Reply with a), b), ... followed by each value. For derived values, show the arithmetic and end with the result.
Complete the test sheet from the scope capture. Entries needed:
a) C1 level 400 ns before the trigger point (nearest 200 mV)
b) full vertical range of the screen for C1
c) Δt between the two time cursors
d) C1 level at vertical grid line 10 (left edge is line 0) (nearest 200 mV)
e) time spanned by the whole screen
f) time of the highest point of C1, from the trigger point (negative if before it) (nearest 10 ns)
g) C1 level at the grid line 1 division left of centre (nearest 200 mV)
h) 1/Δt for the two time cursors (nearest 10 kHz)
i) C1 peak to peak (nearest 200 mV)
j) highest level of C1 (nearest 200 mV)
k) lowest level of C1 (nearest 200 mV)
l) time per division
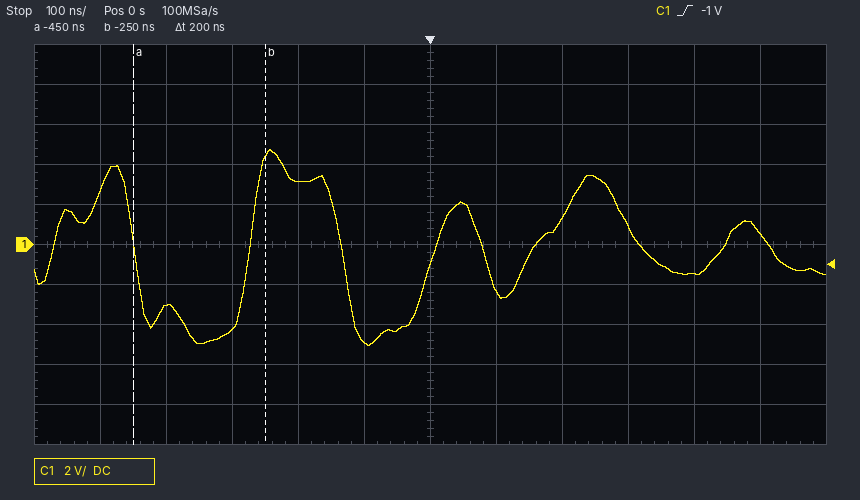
a) -3.0 V
b) 20 V
c) 200 ns
d) -1.4 V
e) 1.2 µs
f) -240 ns
g) -4.8 V
h) 1 / 200 ns ≈ 5.00 MHz
i) 4.8 V − (-5.0 V) = 9.8 V
j) 4.8 V
k) -5.0 V
l) 100 ns
